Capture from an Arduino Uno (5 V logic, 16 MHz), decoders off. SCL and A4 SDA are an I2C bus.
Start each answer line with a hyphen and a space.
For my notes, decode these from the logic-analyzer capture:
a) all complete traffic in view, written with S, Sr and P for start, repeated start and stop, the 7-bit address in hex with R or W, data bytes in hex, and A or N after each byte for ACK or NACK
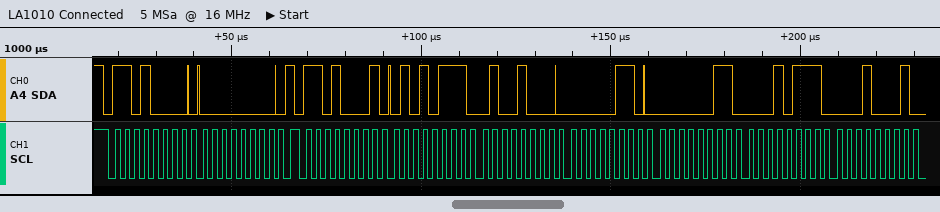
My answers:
- S 68W A 00 A Sr 68R A 57 A 48 A 06 A 03 A 17 A 11 A
